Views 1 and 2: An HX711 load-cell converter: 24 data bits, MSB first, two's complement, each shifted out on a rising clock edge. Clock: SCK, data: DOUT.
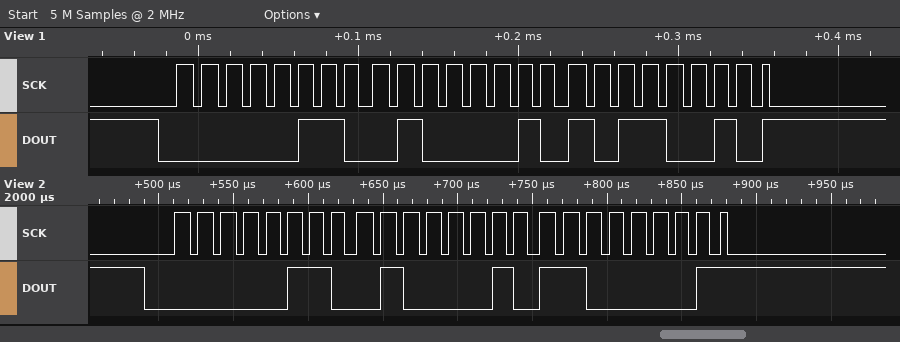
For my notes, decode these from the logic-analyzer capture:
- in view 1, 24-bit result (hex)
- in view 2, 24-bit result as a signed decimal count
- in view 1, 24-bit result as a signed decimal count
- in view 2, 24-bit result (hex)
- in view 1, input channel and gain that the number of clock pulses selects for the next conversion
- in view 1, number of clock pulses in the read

0x0642B2
410305
410290
0x0642C1
channel A, gain 128
25
